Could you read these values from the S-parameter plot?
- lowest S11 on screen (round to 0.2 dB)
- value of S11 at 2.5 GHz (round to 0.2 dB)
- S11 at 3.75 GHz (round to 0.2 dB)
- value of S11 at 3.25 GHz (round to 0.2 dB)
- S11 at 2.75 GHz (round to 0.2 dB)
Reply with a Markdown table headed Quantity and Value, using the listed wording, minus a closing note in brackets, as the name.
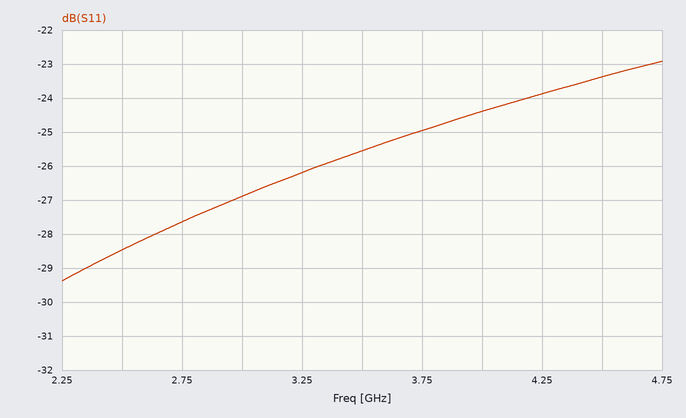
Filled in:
| Quantity | Value |
|---|---|
| lowest S11 on screen | -29.4 dB |
| value of S11 at 2.5 GHz | -28.4 dB |
| S11 at 3.75 GHz | -25.0 dB |
| value of S11 at 3.25 GHz | -26.2 dB |
| S11 at 2.75 GHz | -27.6 dB |
